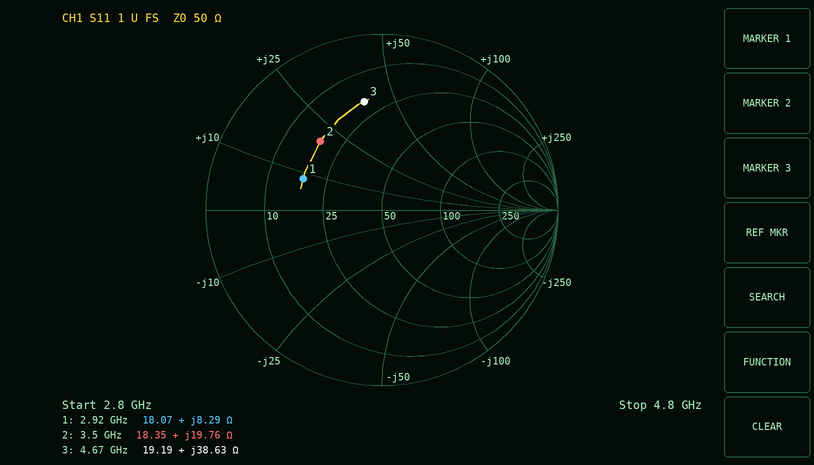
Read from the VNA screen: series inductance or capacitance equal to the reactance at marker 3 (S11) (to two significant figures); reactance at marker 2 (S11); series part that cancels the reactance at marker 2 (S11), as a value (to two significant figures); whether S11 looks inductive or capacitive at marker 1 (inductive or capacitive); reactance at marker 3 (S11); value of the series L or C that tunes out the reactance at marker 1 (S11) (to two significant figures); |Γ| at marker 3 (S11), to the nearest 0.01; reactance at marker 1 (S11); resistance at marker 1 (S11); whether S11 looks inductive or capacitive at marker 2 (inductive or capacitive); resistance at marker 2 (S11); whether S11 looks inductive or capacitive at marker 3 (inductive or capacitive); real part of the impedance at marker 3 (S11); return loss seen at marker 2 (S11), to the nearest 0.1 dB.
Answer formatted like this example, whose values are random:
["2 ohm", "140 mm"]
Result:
["1.3 nH", "+19.76 Ω", "2.3 pF", "inductive", "+38.63 Ω", "6.6 pF", "0.62", "+8.29 Ω", "18.07 Ω", "inductive", "18.35 Ω", "inductive", "19.19 Ω", "5.6 dB"]
